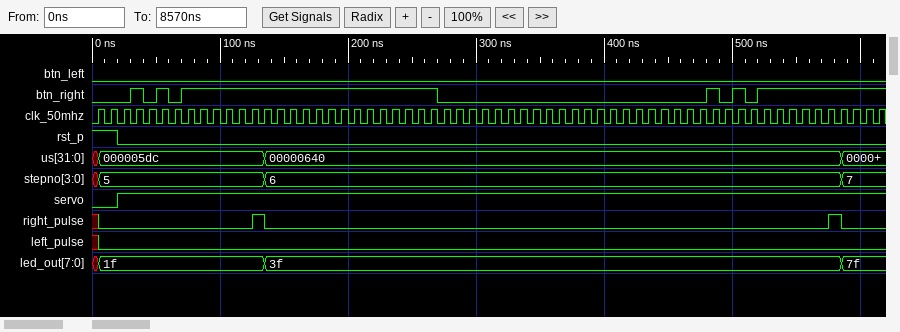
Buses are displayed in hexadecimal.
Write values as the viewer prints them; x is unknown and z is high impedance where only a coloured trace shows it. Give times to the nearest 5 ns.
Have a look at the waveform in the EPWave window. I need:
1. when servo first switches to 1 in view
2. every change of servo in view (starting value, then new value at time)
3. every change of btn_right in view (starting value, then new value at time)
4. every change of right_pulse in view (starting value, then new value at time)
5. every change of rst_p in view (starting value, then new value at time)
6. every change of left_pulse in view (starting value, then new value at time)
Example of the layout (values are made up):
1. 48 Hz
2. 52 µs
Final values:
1. 20 ns
2. 0, 1 at 20 ns
3. 0, 1 at 30 ns, 0 at 40 ns, 1 at 50 ns, 0 at 60 ns, 1 at 70 ns, 0 at 270 ns, 1 at 480 ns, 0 at 490 ns, 1 at 500 ns, 0 at 510 ns, 1 at 520 ns
4. x, 0 at 5 ns, 1 at 125 ns, 0 at 135 ns, 1 at 575 ns, 0 at 585 ns
5. 1, 0 at 20 ns
6. x, 0 at 5 ns
